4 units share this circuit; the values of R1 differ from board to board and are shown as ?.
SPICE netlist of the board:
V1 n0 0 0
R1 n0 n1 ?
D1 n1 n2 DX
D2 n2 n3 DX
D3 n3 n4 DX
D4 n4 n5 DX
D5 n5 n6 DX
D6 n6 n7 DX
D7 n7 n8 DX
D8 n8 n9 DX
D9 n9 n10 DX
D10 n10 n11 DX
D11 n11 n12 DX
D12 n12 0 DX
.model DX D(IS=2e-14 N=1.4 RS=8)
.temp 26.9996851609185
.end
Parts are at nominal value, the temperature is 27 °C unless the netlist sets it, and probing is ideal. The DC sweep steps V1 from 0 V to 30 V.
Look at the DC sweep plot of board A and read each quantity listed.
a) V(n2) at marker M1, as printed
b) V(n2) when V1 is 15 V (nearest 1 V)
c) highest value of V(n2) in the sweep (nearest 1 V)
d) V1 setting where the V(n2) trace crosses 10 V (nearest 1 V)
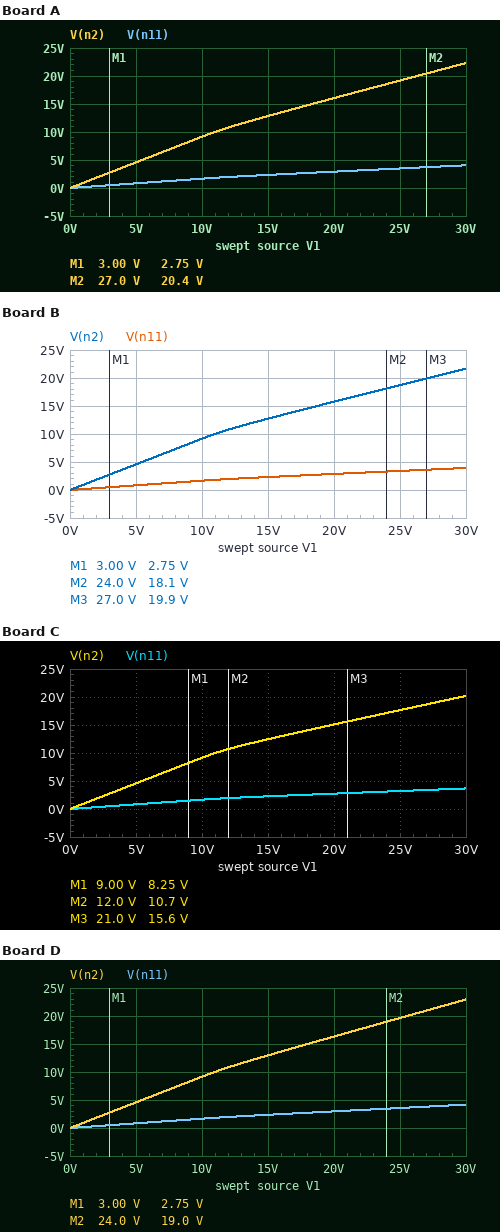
2.75 V
13 V
22 V
11 V
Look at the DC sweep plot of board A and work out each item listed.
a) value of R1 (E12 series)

47 Ω
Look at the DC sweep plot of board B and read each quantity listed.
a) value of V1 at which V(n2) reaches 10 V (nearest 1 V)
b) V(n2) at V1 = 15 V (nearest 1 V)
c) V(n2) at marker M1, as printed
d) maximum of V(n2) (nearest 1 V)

11 V
13 V
2.75 V
22 V
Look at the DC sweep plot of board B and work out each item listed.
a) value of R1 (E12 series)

56 Ω
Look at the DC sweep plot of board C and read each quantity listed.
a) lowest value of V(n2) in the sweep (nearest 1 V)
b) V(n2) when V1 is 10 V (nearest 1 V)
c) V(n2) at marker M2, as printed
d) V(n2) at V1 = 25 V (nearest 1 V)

0 V
9 V
10.7 V
18 V
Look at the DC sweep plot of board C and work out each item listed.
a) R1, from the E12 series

82 Ω
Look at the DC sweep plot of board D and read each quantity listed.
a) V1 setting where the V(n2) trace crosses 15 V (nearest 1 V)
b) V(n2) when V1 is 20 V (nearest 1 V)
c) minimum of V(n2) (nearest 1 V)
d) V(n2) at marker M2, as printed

18 V
16 V
0 V
19.0 V
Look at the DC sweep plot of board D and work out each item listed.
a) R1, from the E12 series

39 Ω
